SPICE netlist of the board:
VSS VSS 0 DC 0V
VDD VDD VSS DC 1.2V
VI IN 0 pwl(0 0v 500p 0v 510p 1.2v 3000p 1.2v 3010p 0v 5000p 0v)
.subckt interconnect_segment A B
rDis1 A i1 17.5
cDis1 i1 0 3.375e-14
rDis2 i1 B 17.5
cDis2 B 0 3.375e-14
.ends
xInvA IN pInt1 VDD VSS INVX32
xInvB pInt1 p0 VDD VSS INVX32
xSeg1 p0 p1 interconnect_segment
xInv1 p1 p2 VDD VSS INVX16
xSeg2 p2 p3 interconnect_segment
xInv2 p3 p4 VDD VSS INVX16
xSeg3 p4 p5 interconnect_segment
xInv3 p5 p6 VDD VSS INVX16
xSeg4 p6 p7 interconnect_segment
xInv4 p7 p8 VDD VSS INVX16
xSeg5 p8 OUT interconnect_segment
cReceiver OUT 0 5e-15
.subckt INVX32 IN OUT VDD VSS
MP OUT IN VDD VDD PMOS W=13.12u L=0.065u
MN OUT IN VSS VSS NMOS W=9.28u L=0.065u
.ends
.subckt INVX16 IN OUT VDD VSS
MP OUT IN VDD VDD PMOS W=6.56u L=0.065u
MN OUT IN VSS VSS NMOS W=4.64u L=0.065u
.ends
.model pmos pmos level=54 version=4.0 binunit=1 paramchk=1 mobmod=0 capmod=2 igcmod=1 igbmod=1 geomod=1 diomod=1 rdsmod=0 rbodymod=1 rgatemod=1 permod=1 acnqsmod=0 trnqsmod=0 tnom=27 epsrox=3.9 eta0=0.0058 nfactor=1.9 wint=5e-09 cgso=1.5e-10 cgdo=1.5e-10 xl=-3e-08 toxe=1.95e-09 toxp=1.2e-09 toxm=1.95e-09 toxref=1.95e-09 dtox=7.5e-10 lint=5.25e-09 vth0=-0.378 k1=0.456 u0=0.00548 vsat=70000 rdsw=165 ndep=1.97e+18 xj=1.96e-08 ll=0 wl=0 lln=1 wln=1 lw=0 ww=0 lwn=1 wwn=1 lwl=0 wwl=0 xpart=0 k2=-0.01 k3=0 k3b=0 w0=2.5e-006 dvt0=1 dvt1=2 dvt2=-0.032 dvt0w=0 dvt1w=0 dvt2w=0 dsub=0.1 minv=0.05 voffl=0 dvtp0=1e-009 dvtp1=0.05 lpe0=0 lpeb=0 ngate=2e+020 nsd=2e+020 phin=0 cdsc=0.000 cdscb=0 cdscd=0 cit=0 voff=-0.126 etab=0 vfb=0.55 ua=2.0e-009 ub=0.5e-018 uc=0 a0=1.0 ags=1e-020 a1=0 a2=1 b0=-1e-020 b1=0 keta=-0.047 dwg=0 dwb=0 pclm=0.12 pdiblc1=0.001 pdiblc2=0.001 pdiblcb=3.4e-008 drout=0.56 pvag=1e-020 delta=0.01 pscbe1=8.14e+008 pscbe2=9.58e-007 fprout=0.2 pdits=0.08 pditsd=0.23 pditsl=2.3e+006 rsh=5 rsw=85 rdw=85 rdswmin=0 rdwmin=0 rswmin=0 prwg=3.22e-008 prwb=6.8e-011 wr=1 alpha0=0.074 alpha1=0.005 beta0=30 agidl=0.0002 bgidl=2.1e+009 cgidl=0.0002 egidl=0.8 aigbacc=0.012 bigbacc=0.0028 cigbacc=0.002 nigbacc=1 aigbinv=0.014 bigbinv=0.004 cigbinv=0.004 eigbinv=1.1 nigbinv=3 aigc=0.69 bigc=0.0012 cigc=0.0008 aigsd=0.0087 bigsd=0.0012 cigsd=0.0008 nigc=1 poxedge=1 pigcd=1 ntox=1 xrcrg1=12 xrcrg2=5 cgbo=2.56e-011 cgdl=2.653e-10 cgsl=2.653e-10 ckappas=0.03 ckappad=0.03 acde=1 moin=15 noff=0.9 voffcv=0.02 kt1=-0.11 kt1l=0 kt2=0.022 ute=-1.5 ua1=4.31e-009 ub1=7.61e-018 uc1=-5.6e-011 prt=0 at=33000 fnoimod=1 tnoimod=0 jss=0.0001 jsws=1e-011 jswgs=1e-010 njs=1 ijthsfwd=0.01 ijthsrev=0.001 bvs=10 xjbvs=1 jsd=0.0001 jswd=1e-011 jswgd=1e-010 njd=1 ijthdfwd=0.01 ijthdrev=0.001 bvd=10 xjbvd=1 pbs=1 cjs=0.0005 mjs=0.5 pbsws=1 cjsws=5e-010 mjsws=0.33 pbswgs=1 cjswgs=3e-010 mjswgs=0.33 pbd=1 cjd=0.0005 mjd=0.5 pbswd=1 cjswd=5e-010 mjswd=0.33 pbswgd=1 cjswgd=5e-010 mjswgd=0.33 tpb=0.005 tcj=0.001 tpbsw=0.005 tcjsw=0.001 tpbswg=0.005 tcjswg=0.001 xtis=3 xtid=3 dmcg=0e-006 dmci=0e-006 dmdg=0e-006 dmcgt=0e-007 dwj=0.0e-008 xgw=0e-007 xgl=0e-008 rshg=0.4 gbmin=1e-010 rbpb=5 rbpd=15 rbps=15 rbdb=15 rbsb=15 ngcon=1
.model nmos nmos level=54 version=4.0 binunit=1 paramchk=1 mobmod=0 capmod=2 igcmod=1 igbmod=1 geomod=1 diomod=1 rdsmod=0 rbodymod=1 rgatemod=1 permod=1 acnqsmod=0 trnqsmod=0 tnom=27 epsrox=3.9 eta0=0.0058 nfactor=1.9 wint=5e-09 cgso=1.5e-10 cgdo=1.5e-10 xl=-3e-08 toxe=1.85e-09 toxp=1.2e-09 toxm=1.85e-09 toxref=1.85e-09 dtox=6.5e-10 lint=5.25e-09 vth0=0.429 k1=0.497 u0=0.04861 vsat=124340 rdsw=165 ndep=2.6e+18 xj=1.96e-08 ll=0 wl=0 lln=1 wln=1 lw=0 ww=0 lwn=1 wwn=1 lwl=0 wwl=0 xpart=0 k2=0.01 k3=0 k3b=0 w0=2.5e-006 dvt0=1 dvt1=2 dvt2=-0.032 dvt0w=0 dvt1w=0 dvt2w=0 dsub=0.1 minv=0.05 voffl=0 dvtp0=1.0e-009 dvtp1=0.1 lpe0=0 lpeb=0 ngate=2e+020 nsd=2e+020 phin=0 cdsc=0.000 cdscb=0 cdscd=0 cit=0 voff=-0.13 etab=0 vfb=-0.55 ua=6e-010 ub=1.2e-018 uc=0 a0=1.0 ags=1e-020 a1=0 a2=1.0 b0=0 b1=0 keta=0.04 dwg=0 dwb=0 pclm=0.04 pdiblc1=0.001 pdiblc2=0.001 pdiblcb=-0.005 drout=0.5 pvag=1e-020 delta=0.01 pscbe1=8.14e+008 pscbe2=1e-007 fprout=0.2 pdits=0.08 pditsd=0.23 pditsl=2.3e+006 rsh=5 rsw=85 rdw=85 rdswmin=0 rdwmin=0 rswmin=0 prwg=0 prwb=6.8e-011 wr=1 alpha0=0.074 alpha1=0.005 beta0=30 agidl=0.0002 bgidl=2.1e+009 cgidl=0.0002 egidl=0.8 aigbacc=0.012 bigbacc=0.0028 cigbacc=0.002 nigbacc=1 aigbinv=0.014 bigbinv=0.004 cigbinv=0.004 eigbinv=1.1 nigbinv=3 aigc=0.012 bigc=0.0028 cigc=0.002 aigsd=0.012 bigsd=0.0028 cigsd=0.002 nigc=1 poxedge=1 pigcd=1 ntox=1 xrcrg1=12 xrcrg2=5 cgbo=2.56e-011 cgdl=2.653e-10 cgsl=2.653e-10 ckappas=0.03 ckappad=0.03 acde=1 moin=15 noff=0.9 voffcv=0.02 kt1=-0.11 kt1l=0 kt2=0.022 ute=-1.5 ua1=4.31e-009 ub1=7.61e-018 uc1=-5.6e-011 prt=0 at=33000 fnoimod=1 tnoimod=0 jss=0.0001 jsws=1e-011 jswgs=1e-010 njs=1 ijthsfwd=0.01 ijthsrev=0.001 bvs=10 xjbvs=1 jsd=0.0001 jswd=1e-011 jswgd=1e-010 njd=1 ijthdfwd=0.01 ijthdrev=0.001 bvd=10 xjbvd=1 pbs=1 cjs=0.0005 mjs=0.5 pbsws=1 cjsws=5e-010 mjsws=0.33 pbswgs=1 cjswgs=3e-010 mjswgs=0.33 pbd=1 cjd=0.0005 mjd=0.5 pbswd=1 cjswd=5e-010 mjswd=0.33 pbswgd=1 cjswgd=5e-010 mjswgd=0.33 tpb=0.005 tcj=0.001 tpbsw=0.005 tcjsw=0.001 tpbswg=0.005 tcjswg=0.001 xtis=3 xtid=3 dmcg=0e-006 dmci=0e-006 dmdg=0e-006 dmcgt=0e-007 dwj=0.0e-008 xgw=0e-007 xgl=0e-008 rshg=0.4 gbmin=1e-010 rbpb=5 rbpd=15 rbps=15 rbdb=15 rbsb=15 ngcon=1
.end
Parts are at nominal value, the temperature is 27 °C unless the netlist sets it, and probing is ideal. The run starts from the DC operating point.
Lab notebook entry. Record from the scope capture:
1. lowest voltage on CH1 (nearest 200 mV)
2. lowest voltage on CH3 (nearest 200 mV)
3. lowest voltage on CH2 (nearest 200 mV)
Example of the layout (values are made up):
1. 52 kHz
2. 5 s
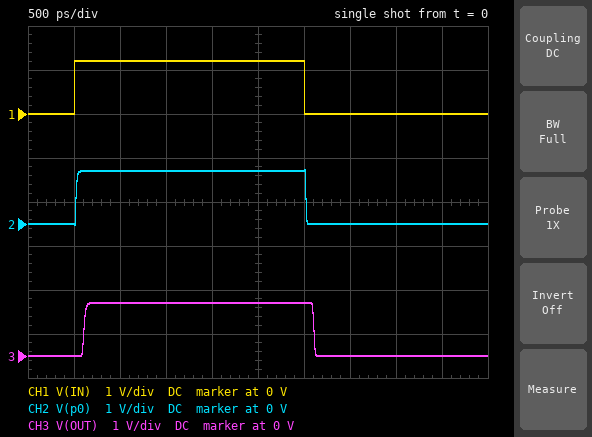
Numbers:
1. 0 V
2. 0 V
3. 0 V
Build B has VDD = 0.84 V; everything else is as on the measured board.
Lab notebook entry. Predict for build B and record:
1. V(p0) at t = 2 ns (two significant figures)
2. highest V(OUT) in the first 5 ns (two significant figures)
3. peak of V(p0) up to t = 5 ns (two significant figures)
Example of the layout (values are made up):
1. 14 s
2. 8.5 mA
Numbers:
1. 840 mV
2. 850 mV
3. 870 mV
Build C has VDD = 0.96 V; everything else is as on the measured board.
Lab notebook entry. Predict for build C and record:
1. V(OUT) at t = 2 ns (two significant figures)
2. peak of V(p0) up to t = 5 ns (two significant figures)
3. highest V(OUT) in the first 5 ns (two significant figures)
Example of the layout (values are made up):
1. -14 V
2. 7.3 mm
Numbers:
1. 960 mV
2. 990 mV
3. 970 mV
